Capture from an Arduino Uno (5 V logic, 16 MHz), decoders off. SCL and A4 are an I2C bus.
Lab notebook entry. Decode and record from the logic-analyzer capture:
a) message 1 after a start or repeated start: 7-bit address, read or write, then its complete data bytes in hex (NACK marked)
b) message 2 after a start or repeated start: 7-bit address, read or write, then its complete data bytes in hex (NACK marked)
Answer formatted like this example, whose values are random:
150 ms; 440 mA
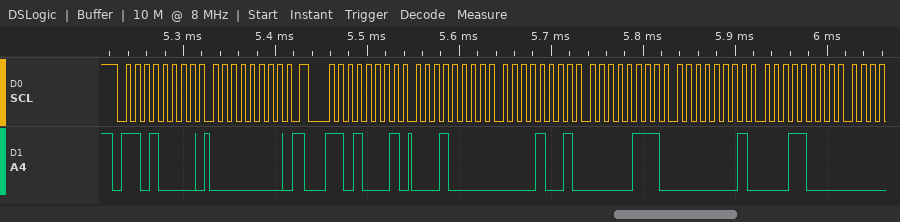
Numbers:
0x68 write: 00; 0x68 read: 10 09 07 01 18
